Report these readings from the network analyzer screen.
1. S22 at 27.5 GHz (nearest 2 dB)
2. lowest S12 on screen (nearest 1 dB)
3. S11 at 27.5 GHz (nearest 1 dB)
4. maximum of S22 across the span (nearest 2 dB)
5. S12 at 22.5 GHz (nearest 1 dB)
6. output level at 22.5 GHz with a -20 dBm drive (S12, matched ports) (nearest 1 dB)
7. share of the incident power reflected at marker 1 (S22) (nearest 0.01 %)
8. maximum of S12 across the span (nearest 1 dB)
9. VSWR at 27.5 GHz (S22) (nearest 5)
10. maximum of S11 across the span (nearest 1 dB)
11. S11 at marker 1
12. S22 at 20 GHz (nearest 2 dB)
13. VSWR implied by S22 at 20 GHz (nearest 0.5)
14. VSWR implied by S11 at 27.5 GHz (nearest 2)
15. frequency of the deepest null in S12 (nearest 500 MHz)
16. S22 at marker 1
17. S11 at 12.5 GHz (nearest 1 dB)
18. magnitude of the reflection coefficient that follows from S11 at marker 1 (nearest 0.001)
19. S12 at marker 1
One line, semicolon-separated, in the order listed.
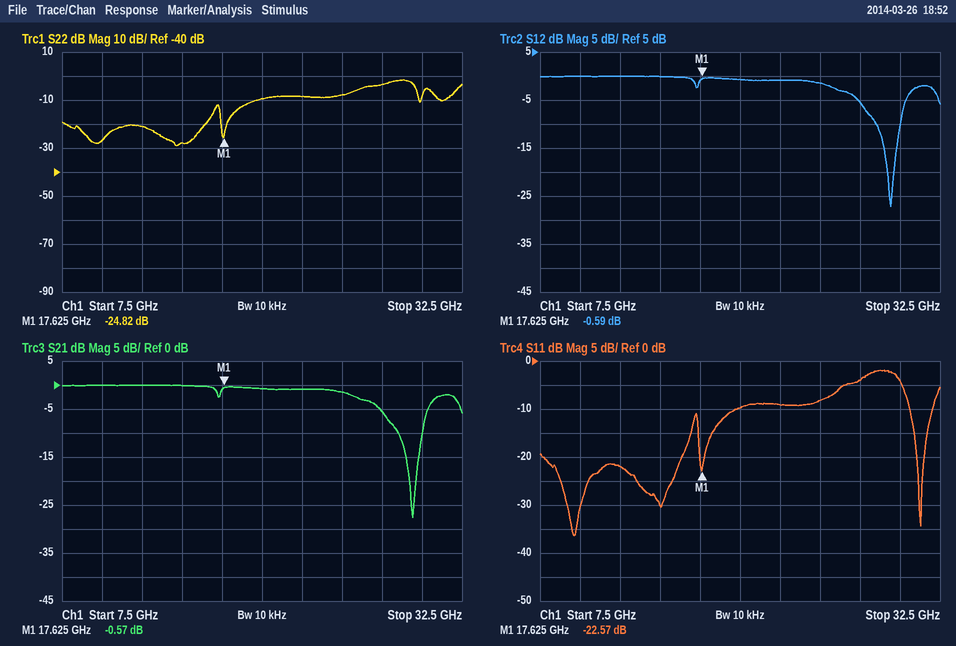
-4 dB; -27 dB; -4 dB; -2 dB; -1 dB; -21 dBm; 0.33 %; 0 dB; 5; -2 dB; -22.57 dB; -10 dB; 2.0; 4; 29.5 GHz; -24.82 dB; -22 dB; 0.074; -0.59 dB
